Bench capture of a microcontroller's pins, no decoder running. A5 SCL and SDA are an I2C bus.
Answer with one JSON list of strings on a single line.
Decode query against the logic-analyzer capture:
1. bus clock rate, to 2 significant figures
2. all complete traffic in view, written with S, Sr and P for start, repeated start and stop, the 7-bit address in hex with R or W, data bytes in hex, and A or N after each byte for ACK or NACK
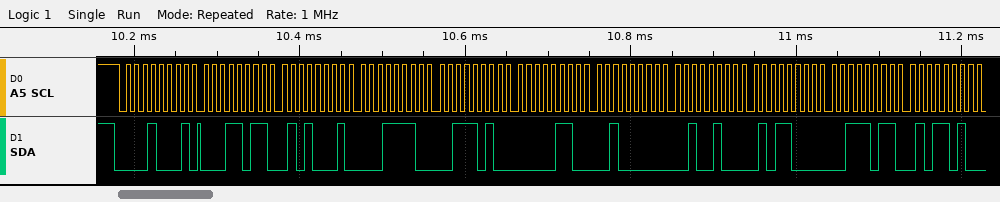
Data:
["100 kHz", "S 08R A 1B A 51 A 1E A 3A A 06 A 20 A 24 A 58 A 3B A 5A A"]
